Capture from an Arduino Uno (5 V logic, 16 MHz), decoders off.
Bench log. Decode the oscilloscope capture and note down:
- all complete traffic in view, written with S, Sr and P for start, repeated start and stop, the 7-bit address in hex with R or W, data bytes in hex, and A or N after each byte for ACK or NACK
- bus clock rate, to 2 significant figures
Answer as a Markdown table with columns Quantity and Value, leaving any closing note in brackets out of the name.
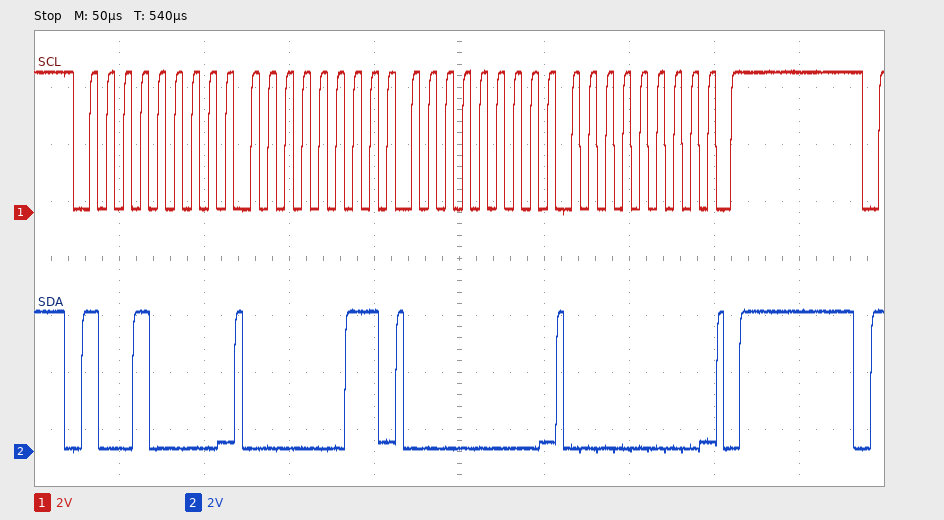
| Quantity | Value |
|---|---|
| all complete traffic in view, written with S, Sr and P for start, repeated start and stop, the 7-bit address in hex with R or W, data bytes in hex, and A or N after each byte for ACK or NACK | S 48W A 03 A 00 A 00 A P |
| bus clock rate, to 2 significant figures | 100 kHz |
